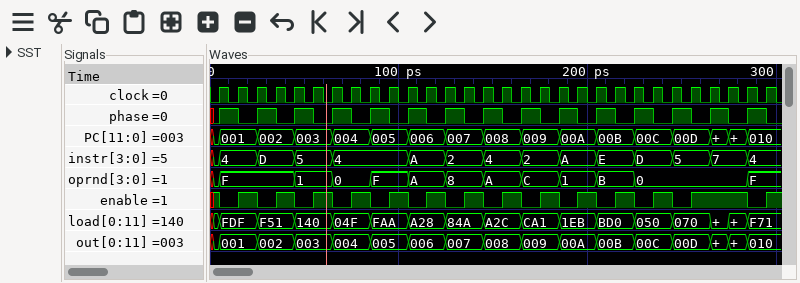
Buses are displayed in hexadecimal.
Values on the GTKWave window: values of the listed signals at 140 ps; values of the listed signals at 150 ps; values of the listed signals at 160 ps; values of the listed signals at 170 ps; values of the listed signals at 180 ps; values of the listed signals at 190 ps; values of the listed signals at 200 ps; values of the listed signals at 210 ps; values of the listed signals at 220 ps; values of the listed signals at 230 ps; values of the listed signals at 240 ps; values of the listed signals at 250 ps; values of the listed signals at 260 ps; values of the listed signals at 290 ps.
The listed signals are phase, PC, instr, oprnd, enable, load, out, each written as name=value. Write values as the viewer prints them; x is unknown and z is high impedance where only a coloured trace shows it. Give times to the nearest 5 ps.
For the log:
phase=0, PC=007, instr=2, oprnd=8, enable=1, load=84A, out=007
phase=1, PC=008, instr=4, oprnd=A, enable=0, load=A2C, out=008
phase=0, PC=008, instr=4, oprnd=A, enable=1, load=A2C, out=008
phase=1, PC=009, instr=2, oprnd=C, enable=0, load=CA1, out=009
phase=0, PC=009, instr=2, oprnd=C, enable=1, load=CA1, out=009
phase=1, PC=00A, instr=A, oprnd=1, enable=0, load=1EB, out=00A
phase=0, PC=00A, instr=A, oprnd=1, enable=1, load=1EB, out=00A
phase=1, PC=00B, instr=E, oprnd=B, enable=0, load=BD0, out=00B
phase=0, PC=00B, instr=E, oprnd=B, enable=1, load=BD0, out=00B
phase=1, PC=00C, instr=D, oprnd=0, enable=0, load=050, out=00C
phase=0, PC=00C, instr=D, oprnd=0, enable=1, load=050, out=00C
phase=1, PC=00D, instr=5, oprnd=0, enable=0, load=070, out=00D
phase=0, PC=00D, instr=5, oprnd=0, enable=1, load=070, out=00D
phase=1, PC=010, instr=4, oprnd=F, enable=0, load=F71, out=010
